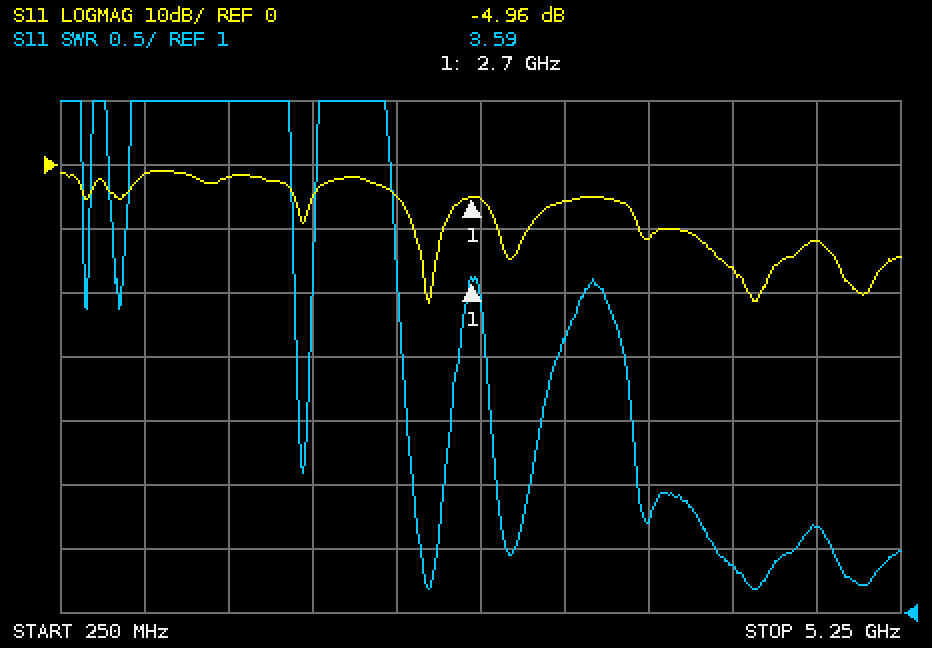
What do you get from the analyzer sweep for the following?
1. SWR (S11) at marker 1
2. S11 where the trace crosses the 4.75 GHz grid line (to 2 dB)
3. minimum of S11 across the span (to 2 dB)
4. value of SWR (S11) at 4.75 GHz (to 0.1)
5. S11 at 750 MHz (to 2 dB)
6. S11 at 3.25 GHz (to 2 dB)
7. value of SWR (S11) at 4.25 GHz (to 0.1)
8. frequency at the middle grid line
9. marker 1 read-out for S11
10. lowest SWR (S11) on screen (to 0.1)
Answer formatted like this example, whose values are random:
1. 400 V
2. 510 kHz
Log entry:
1. 3.59
2. -12 dB
3. -22 dB
4. 1.7
5. -2 dB
6. -6 dB
7. 1.4
8. 2.75 GHz
9. -4.96 dB
10. 1.2
